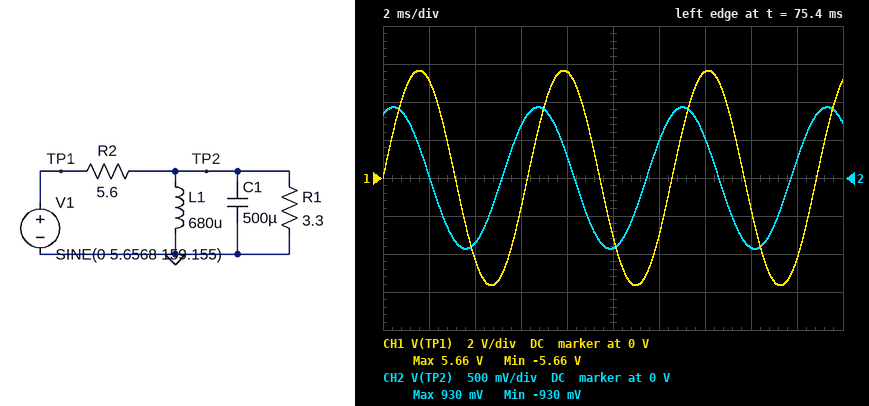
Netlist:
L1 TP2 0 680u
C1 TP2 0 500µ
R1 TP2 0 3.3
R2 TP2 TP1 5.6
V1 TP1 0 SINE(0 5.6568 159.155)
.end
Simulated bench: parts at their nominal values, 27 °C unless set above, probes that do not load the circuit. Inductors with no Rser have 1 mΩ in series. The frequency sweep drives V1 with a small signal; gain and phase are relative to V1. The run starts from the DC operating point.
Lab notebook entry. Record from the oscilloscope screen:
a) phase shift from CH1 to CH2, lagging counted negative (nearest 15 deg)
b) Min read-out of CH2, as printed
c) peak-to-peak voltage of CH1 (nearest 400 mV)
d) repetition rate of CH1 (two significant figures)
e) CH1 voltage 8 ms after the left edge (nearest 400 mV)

60 deg
-930 mV
11.2 V
160 Hz
5.6 V
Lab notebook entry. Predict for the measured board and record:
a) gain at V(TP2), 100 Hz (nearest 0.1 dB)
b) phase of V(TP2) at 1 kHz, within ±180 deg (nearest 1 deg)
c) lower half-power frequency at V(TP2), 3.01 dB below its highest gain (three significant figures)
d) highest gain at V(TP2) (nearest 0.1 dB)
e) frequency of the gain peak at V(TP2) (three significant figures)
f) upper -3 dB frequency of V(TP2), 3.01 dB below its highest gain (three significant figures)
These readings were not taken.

-21.3 dB
-81 deg
207 Hz
-8.6 dB
273 Hz
360 Hz
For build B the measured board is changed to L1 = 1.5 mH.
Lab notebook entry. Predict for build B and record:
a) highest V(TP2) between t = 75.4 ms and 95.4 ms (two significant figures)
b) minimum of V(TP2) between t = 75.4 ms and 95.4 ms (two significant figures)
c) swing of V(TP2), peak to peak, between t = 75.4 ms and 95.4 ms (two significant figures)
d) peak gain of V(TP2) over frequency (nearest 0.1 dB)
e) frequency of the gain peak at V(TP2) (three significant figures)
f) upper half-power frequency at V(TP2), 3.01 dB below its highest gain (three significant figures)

2.0 V
-2.0 V
4.0 V
-8.6 dB
184 Hz
276 Hz
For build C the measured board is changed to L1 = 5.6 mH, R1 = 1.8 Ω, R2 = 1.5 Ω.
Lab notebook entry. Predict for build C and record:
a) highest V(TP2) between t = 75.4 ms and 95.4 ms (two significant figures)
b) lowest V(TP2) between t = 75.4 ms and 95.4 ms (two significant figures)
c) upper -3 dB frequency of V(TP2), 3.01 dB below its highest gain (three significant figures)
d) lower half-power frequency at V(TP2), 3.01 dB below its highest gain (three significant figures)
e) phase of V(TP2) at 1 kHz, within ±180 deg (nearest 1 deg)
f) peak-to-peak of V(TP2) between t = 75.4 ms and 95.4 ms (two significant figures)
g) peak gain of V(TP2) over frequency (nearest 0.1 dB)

3.0 V
-3.0 V
411 Hz
22.0 Hz
-69 deg
6.0 V
-5.3 dB
